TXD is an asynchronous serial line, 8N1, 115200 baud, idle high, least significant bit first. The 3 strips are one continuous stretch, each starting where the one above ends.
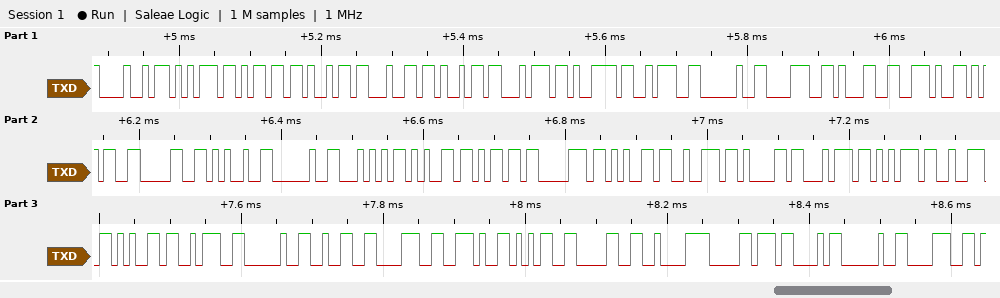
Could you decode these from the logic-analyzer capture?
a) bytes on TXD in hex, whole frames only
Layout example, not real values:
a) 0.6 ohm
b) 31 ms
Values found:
a) 48 75 6D 69 64 69 74 79 3A 20 38 31 2E 35 30 25 20 54 65 6D 70 65 72 61 74 75 72 65 3A 20 32 38 2E 35 30 C2 B0 43 20 38
